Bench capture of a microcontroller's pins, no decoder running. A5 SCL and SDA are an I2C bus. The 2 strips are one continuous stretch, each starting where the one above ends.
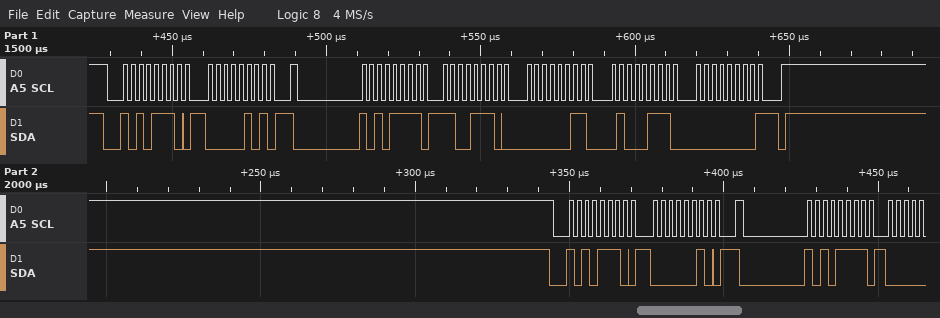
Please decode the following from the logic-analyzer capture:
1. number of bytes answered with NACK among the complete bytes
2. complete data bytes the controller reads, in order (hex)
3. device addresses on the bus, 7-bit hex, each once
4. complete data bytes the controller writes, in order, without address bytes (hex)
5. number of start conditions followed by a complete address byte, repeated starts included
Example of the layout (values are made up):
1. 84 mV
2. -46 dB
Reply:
1. 1
2. CE 03 47 00
3. 0x57
4. 05 02
5. 4
